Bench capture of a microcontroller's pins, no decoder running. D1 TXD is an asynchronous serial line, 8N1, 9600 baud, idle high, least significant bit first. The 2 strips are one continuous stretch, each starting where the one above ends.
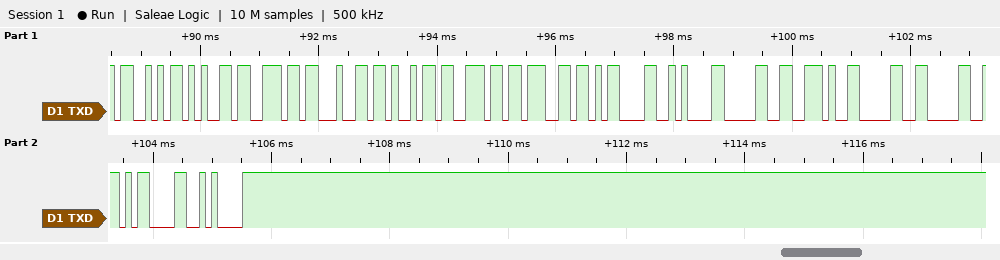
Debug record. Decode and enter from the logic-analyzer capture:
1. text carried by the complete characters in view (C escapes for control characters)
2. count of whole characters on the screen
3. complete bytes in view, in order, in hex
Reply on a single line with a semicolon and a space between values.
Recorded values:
"Sending\r\n0.00\r\n"; 15; 0x53 0x65 0x6E 0x64 0x69 0x6E 0x67 0x0D 0x0A 0x30 0x2E 0x30 0x30 0x0D 0x0A
